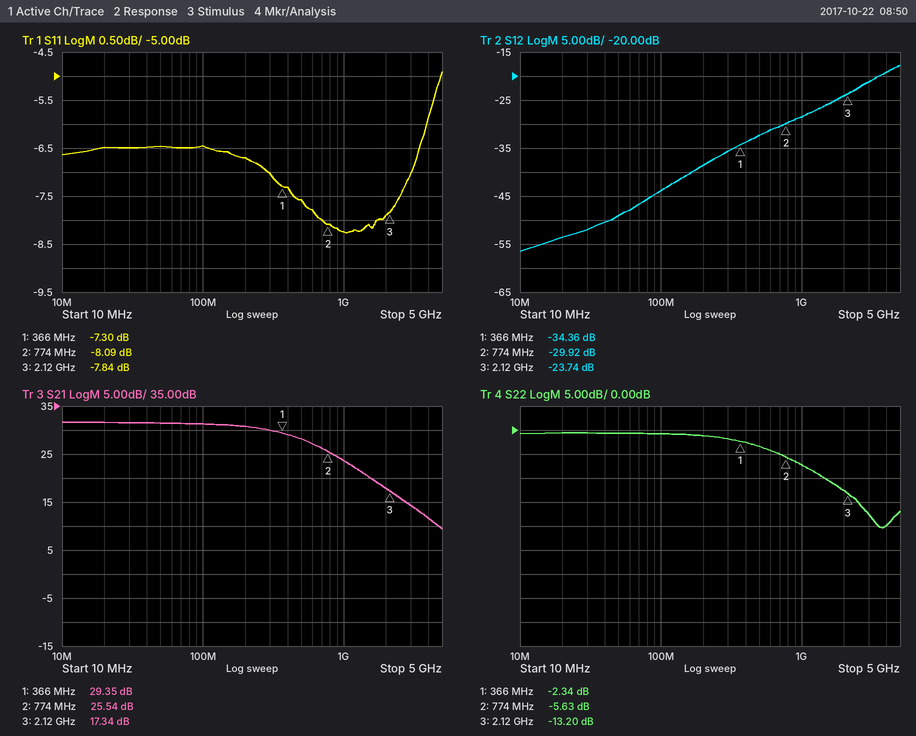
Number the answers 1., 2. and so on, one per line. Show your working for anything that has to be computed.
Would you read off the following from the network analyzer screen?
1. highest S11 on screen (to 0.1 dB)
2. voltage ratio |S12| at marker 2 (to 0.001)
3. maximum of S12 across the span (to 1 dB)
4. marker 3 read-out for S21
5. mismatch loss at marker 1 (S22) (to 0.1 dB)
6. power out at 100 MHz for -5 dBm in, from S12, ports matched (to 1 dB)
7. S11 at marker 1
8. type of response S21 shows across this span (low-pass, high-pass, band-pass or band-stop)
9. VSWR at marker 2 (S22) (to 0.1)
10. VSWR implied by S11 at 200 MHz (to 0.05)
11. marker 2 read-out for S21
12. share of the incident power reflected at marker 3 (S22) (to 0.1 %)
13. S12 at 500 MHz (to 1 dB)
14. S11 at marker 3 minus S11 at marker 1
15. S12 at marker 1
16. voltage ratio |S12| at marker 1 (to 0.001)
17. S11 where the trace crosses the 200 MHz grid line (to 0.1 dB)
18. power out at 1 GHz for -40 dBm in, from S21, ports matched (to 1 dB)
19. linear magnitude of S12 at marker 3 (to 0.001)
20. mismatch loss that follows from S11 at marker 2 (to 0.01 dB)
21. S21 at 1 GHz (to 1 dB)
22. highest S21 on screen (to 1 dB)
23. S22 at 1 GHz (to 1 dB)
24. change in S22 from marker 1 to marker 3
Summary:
1. -4.9 dB
2. 10^(-29.92/20) ≈ 0.032
3. -18 dB
4. 17.34 dB
5. −10 log10(1 − 10^(-2.34/10)) ≈ 3.8 dB
6. -5 dBm + (-44 dB) = -49 dBm
7. -7.30 dB
8. low-pass
9. (1 + 0.5230)/(1 − 0.5230) ≈ 3.2
10. |Γ| = 10^(-6.7/20) = 0.4624; VSWR = (1 + 0.4624)/(1 − 0.4624) ≈ 2.72, so 2.70 to the nearest 0.05
11. 25.54 dB
12. 10^(-13.2/10) ≈ 4.8 %
13. -32 dB
14. -7.84 − (-7.3) = -0.54 dB
15. -34.36 dB
16. 10^(-34.36/20) ≈ 0.019
17. -6.7 dB
18. -40 dBm + (24 dB) = -16 dBm
19. 10^(-23.74/20) ≈ 0.065
20. −10 log10(1 − 10^(-8.09/10)) ≈ 0.73 dB
21. 24 dB
22. 32 dB
23. -7 dB
24. -13.2 − (-2.34) = -10.86 dB
